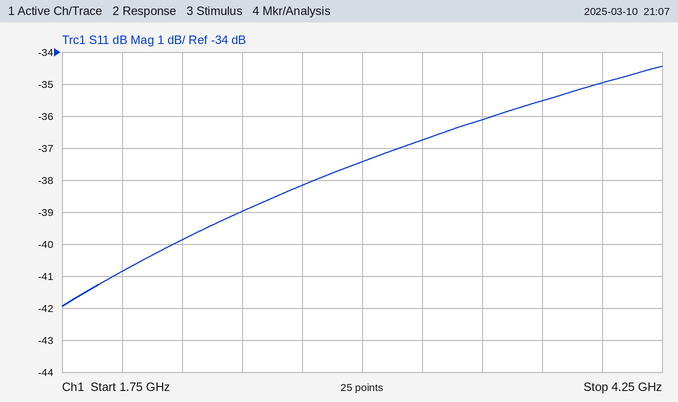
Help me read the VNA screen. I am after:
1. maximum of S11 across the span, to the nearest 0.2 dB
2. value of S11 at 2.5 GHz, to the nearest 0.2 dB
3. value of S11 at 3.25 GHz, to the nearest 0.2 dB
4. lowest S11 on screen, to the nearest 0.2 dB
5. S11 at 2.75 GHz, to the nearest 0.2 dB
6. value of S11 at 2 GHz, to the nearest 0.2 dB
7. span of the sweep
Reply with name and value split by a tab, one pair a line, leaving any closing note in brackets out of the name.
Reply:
maximum of S11 across the span, to the nearest 0.2 dB	-34.4 dB
value of S11 at 2.5 GHz, to the nearest 0.2 dB	-39.0 dB
value of S11 at 3.25 GHz, to the nearest 0.2 dB	-36.8 dB
lowest S11 on screen, to the nearest 0.2 dB	-42.0 dB
S11 at 2.75 GHz, to the nearest 0.2 dB	-38.2 dB
value of S11 at 2 GHz, to the nearest 0.2 dB	-40.8 dB
span of the sweep	2.5 GHz
